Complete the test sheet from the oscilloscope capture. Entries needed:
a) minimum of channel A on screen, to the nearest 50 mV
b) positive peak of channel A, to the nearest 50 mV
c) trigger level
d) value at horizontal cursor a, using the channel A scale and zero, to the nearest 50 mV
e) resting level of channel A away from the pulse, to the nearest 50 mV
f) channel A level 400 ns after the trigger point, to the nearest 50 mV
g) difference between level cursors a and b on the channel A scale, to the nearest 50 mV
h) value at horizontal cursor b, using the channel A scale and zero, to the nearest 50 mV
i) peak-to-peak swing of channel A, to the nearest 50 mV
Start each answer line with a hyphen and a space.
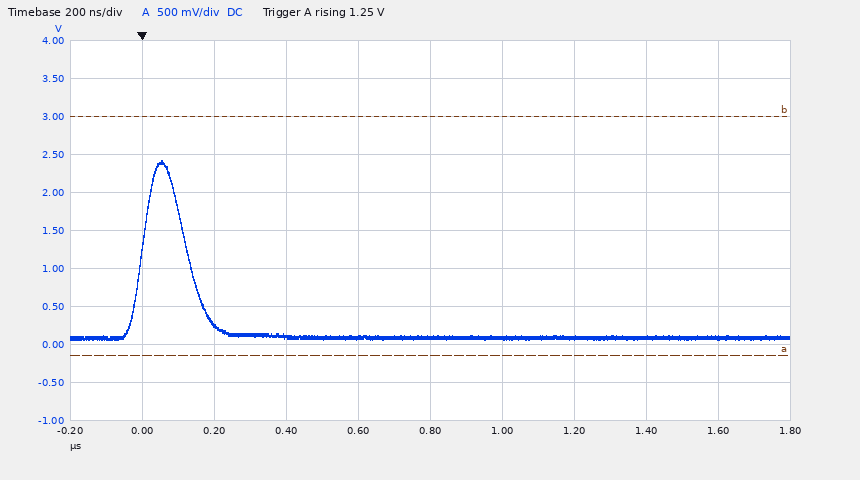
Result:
- 50 mV
- 2.40 V
- 1.25 V
- -150 mV
- 100 mV
- 100 mV
- 3.15 V
- 3.00 V
- 2.35 V
